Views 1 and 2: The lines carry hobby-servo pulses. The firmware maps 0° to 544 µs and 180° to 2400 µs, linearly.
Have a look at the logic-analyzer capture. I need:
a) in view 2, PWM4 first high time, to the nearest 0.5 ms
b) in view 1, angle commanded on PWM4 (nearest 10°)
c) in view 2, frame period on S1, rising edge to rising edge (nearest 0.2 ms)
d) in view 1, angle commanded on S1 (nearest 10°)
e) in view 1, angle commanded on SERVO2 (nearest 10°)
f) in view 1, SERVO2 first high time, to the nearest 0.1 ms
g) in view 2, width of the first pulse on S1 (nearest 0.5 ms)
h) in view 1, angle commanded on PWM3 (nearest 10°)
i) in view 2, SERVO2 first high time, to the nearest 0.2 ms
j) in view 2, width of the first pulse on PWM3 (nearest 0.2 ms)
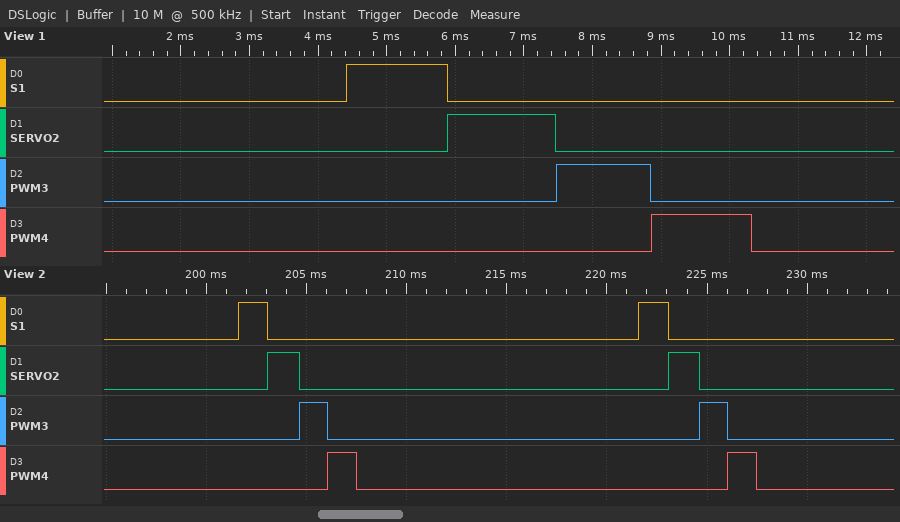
1.5 ms
90°
20.0 ms
90°
100°
1.6 ms
1.5 ms
80°
1.6 ms
1.4 ms
